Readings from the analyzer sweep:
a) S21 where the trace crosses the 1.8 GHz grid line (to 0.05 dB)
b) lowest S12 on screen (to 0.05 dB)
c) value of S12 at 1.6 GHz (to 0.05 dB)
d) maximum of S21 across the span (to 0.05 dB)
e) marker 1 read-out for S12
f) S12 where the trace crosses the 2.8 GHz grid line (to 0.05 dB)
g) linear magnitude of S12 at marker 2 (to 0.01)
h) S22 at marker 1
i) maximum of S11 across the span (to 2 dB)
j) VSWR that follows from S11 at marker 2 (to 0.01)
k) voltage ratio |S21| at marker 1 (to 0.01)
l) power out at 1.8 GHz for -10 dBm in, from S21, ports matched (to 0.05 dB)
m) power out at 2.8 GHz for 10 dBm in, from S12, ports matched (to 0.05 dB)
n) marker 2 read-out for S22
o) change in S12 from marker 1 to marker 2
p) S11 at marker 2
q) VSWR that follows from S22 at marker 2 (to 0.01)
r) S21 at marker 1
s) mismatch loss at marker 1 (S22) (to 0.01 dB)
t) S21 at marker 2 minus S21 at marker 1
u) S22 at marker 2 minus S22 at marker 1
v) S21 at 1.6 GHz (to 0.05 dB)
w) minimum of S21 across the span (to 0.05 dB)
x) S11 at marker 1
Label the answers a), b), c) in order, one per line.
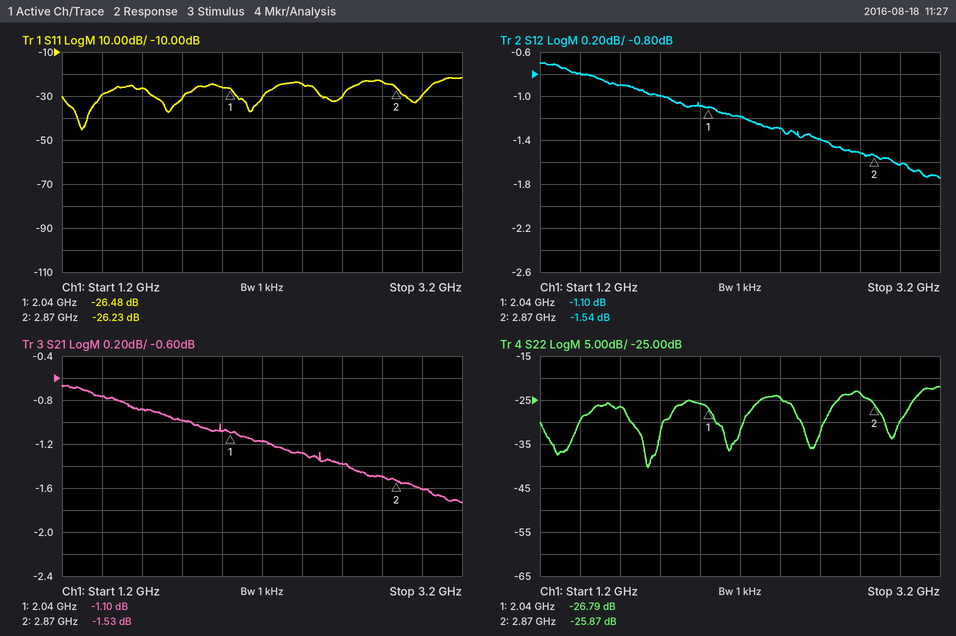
a) -1.00 dB
b) -1.75 dB
c) -0.90 dB
d) -0.65 dB
e) -1.10 dB
f) -1.50 dB
g) 0.84
h) -26.79 dB
i) -22 dB
j) 1.10
k) 0.88
l) -11.00 dBm
m) 8.50 dBm
n) -25.87 dB
o) -0.44 dB
p) -26.23 dB
q) 1.11
r) -1.10 dB
s) 0.01 dB
t) -0.43 dB
u) 0.92 dB
v) -0.90 dB
w) -1.75 dB
x) -26.48 dB
